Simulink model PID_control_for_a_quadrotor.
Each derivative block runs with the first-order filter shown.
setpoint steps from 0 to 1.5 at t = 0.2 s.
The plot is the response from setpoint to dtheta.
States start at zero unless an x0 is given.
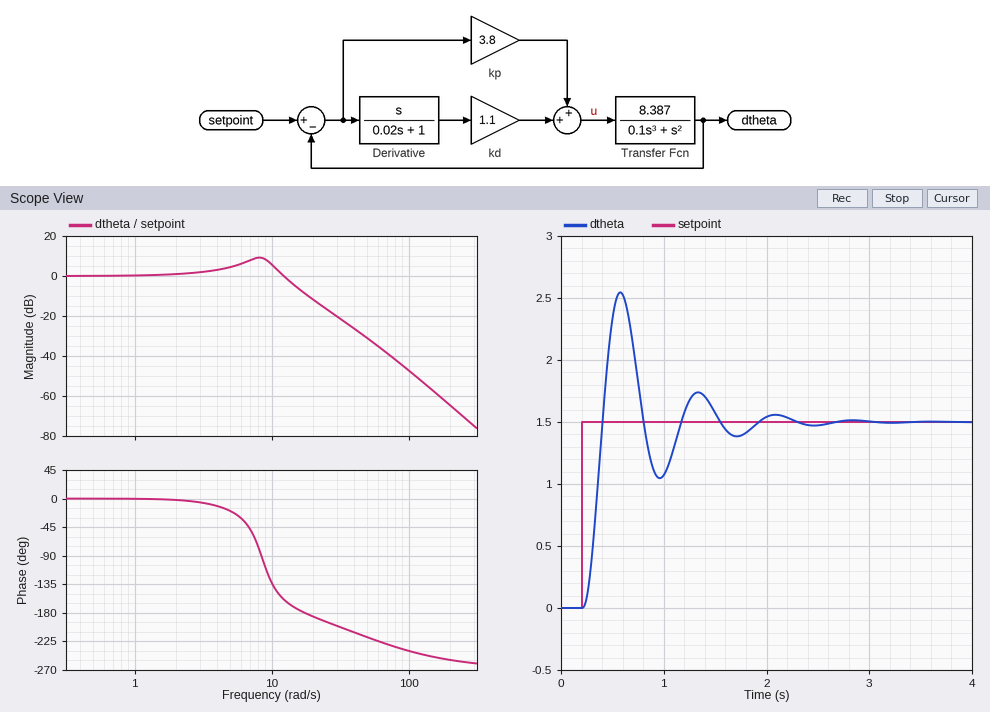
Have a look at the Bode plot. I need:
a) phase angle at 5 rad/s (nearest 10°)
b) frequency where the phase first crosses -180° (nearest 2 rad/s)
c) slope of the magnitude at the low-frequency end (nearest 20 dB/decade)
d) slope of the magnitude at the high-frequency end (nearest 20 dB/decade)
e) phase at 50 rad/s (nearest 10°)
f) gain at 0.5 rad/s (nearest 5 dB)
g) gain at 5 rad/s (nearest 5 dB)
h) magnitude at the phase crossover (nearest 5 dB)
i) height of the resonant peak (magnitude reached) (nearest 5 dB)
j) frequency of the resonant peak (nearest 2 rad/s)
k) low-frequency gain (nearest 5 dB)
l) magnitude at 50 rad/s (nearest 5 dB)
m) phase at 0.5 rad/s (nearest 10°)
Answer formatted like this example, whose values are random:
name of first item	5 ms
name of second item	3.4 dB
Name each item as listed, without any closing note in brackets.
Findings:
phase angle at 5 rad/s	-20°
frequency where the phase first crosses -180°	18 rad/s
slope of the magnitude at the low-frequency end	0 dB/decade
slope of the magnitude at the high-frequency end	-60 dB/decade
phase at 50 rad/s	-220°
gain at 0.5 rad/s	0 dB
gain at 5 rad/s	5 dB
magnitude at the phase crossover	-10 dB
height of the resonant peak (magnitude reached)	10 dB
frequency of the resonant peak	8 rad/s
low-frequency gain	0 dB
magnitude at 50 rad/s	-30 dB
phase at 0.5 rad/s	0°
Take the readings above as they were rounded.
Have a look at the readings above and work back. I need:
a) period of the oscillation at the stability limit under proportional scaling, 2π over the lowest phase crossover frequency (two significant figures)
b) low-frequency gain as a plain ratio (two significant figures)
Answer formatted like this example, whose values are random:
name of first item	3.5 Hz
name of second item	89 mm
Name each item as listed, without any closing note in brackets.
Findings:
period of the oscillation at the stability limit under proportional scaling, 2π over the lowest phase crossover frequency	0.35 s
low-frequency gain as a plain ratio	1.0
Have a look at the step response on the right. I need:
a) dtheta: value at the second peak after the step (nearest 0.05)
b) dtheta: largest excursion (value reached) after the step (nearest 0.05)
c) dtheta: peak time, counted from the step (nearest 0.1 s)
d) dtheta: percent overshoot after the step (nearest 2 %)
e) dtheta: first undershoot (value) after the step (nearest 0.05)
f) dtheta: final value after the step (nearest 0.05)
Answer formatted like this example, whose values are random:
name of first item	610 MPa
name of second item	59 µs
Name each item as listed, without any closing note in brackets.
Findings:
dtheta: value at the second peak after the step	1.75
dtheta: largest excursion (value reached) after the step	2.55
dtheta: peak time, counted from the step	0.4 s
dtheta: percent overshoot after the step	70 %
dtheta: first undershoot (value) after the step	1.05
dtheta: final value after the step	1.50
